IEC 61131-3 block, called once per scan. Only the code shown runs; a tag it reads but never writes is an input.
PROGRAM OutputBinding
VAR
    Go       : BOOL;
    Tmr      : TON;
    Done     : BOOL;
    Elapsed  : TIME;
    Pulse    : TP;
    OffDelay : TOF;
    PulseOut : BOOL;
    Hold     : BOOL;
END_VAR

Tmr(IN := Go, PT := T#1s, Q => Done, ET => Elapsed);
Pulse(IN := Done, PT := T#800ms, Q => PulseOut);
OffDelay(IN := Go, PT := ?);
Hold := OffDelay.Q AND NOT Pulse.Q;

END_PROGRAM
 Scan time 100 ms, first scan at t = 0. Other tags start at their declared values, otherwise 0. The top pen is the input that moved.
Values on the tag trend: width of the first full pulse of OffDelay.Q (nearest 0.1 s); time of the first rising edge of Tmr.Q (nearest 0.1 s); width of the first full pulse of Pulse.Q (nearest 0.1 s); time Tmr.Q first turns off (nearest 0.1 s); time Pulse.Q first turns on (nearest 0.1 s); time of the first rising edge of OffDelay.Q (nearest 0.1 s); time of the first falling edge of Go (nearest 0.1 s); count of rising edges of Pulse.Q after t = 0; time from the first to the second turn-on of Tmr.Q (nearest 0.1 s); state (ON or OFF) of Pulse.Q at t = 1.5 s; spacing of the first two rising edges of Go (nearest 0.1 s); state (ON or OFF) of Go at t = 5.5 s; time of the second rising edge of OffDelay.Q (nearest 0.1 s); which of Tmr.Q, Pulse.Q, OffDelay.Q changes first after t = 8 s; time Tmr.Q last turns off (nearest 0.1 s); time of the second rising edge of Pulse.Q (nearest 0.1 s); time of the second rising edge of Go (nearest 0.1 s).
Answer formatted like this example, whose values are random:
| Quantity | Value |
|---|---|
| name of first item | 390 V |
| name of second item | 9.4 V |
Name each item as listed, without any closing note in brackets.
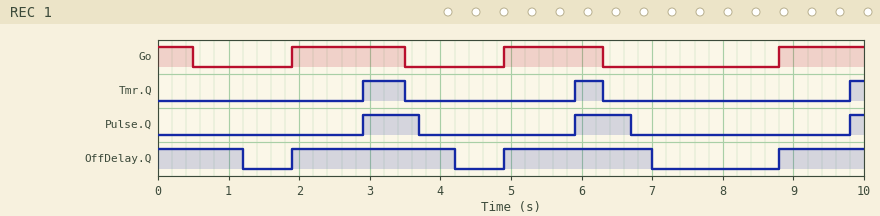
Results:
| Quantity | Value |
|---|---|
| width of the first full pulse of OffDelay.Q | 2.3 s |
| time of the first rising edge of Tmr.Q | 2.9 s |
| width of the first full pulse of Pulse.Q | 0.8 s |
| time Tmr.Q first turns off | 3.5 s |
| time Pulse.Q first turns on | 2.9 s |
| time of the first rising edge of OffDelay.Q | 1.9 s |
| time of the first falling edge of Go | 0.5 s |
| count of rising edges of Pulse.Q after t = 0 | 3 |
| time from the first to the second turn-on of Tmr.Q | 3.0 s |
| state (ON or OFF) of Pulse.Q at t = 1.5 s | OFF |
| spacing of the first two rising edges of Go | 3.0 s |
| state (ON or OFF) of Go at t = 5.5 s | ON |
| time of the second rising edge of OffDelay.Q | 4.9 s |
| which of Tmr.Q, Pulse.Q, OffDelay.Q changes first after t = 8 s | OffDelay.Q |
| time Tmr.Q last turns off | 6.3 s |
| time of the second rising edge of Pulse.Q | 5.9 s |
| time of the second rising edge of Go | 4.9 s |
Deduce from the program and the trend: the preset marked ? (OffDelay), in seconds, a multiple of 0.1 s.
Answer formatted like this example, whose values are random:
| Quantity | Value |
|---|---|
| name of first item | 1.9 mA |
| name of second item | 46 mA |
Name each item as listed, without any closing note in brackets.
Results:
| Quantity | Value |
|---|---|
| the preset marked ? (OffDelay), in seconds, a multiple of 0.1 s | 0.7 s |
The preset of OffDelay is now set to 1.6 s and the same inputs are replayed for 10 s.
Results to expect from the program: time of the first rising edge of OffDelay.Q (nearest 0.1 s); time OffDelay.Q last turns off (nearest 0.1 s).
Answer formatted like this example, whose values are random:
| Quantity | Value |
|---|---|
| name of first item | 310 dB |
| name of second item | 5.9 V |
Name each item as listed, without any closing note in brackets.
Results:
| Quantity | Value |
|---|---|
| time of the first rising edge of OffDelay.Q | 8.8 s |
| time OffDelay.Q last turns off | 7.9 s |
